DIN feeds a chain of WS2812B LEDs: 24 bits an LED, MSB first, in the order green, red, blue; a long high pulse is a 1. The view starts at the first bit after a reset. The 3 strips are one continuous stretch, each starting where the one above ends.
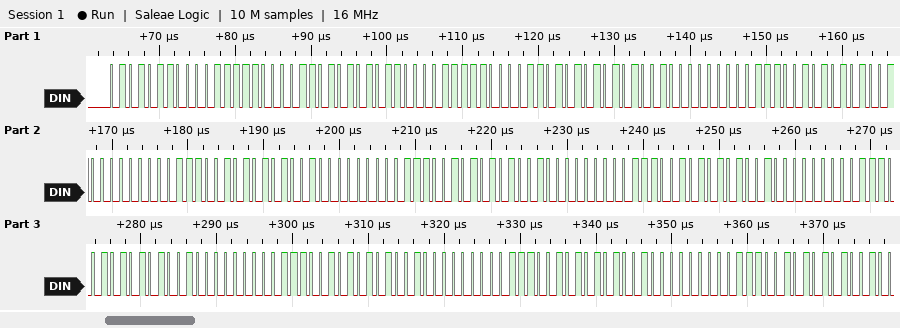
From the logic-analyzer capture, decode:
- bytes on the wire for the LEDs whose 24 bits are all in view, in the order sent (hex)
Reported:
56 1F 0D 56 1F 0D 55 20 0E 55 20 0E 55 20 0E 55 20 0E 55 20 0E 55 20 0E 55 20 0E 55 20 0E
